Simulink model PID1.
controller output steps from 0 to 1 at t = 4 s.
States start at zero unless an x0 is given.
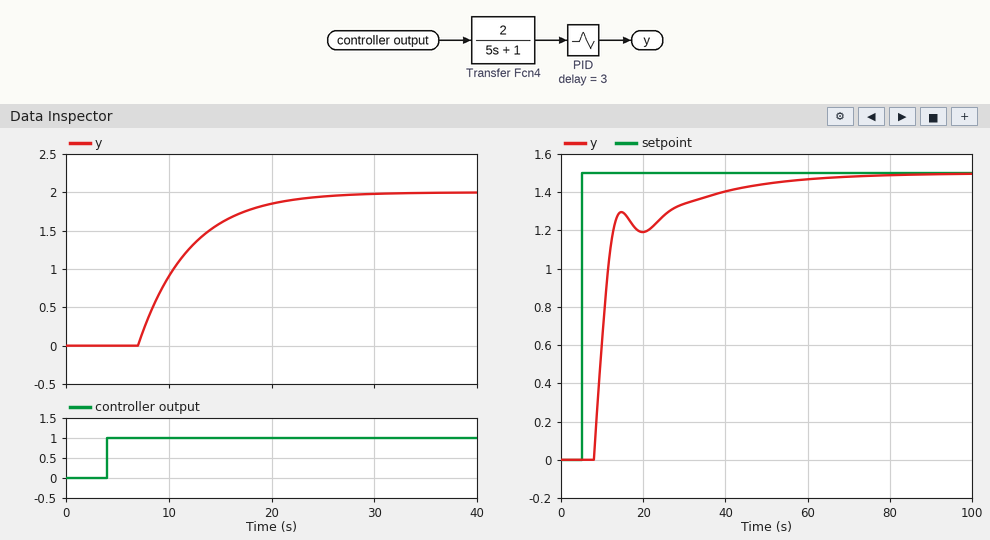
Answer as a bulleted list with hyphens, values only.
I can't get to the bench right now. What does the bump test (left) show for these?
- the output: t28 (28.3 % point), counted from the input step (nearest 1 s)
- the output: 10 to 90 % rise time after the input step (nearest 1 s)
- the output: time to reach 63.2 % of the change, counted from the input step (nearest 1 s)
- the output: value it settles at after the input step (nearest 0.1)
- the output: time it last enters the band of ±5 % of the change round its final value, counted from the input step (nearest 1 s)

- 5 s
- 11 s
- 8 s
- 2.0
- 18 s
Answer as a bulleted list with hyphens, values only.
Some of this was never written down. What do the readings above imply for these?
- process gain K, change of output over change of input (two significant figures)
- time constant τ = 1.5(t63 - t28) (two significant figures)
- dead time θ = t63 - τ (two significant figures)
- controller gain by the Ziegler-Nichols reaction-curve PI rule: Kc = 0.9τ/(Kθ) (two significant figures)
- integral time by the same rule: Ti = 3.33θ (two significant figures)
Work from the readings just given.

- 2.0
- 4.5 s
- 3.5 s
- 0.58
- 12 s
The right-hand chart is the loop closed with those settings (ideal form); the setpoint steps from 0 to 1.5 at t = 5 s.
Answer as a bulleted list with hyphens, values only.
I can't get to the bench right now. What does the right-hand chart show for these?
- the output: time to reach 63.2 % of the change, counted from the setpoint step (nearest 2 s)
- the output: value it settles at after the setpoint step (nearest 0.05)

- 6 s
- 1.50
